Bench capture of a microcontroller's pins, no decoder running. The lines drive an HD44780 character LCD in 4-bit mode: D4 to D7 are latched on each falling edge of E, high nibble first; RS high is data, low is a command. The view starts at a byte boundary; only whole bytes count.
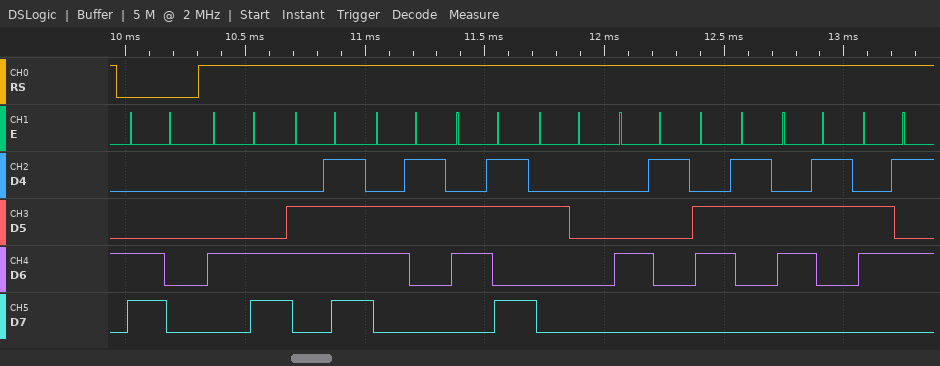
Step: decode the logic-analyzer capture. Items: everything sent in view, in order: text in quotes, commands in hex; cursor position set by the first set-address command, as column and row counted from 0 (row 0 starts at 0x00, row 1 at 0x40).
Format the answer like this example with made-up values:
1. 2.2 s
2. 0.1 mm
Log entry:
1. 0xC0 "Lock Acce"
2. column 0, row 1
